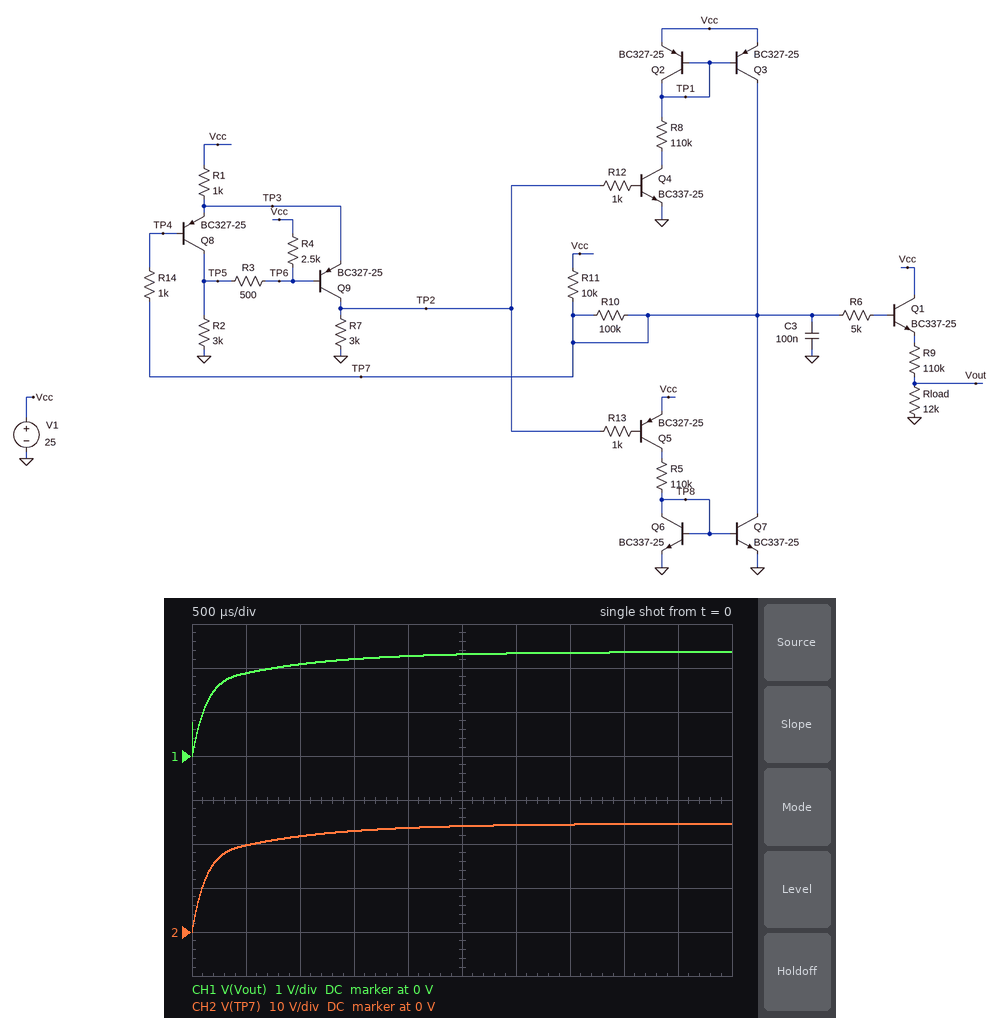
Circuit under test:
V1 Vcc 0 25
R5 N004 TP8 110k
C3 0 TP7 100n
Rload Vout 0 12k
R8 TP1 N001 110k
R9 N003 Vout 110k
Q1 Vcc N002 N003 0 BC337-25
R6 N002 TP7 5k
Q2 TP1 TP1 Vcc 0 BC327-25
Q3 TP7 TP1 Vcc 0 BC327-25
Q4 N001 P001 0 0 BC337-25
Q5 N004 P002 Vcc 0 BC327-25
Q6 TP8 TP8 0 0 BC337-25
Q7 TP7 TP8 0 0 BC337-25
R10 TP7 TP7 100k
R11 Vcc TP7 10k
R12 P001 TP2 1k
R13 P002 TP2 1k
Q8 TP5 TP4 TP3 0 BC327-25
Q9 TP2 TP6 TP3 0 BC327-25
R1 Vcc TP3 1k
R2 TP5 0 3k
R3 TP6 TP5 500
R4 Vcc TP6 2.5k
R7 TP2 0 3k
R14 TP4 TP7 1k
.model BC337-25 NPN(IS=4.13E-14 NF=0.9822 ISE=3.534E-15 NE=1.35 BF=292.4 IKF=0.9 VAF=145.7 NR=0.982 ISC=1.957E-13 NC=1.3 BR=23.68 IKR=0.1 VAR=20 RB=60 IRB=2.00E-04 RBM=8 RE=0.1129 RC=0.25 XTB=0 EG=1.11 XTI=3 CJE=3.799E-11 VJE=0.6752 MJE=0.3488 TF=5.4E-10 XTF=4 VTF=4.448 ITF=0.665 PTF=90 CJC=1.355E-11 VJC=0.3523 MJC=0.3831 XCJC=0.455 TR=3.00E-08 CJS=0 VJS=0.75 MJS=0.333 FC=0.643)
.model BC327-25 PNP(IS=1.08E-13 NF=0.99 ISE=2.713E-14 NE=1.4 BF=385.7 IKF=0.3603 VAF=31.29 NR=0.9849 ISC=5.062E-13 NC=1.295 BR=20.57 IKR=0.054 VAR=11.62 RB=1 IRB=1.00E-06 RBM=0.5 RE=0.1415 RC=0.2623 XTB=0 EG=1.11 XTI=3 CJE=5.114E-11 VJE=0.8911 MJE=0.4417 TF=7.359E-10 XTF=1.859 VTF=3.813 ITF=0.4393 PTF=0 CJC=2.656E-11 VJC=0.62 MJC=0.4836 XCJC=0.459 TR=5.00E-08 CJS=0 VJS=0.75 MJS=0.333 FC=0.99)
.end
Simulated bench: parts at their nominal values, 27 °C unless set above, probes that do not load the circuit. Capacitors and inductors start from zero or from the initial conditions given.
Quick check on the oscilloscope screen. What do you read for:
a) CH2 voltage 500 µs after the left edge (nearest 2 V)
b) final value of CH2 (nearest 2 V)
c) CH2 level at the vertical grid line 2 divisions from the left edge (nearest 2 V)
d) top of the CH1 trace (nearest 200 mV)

20 V
24 V
22 V
2.4 V
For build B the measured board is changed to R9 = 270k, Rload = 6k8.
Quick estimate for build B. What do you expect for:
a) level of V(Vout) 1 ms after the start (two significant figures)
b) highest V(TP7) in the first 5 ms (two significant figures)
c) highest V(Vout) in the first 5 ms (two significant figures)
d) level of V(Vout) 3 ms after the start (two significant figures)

520 mV
25 V
590 mV
580 mV
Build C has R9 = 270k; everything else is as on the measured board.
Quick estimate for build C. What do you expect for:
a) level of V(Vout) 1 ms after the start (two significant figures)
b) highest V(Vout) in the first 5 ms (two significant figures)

900 mV
1.0 V
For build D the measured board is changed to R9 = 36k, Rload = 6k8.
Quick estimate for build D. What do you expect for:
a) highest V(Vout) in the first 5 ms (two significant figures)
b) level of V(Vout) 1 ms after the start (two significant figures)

3.8 V
3.4 V
